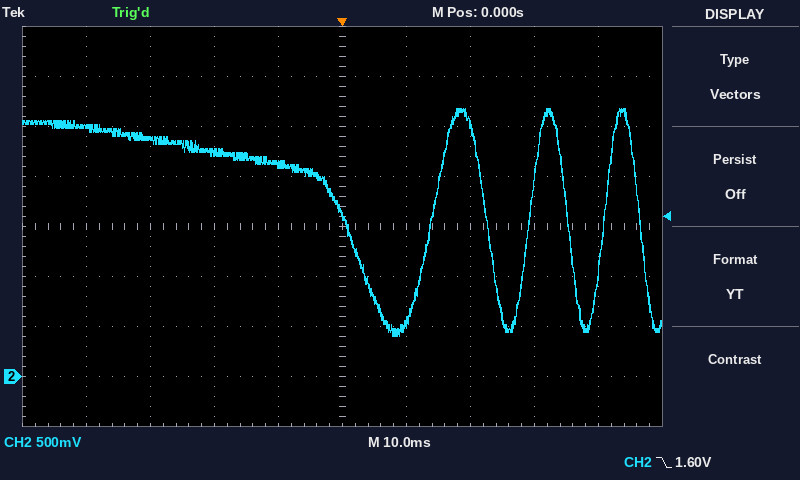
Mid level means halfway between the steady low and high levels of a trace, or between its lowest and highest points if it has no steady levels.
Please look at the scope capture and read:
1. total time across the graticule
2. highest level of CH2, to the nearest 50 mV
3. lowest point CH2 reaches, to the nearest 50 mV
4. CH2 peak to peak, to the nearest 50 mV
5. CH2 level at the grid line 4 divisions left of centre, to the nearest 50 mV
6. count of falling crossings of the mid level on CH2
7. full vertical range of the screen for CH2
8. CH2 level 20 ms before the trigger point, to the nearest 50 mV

100 ms
2.70 V
400 mV
2.30 V
2.50 V
4
4 V
2.25 V
